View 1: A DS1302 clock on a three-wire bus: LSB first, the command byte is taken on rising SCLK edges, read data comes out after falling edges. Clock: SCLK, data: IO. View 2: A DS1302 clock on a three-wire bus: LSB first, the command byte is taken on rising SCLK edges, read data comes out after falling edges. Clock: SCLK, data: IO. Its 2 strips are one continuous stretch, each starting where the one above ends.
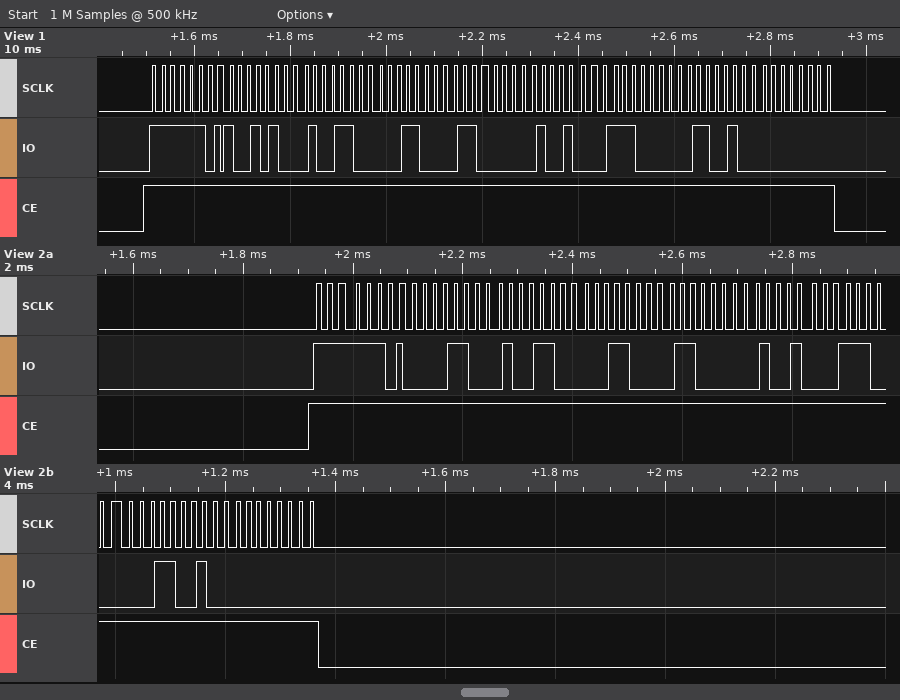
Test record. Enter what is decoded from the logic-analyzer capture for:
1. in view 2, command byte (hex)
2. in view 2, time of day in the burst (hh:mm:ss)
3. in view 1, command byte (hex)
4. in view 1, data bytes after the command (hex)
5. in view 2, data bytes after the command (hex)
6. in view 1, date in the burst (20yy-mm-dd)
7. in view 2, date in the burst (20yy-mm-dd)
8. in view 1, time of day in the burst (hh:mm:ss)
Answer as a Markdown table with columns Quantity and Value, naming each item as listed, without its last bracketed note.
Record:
| Quantity | Value |
|---|---|
| in view 2, command byte | 0xBF |
| in view 2, time of day in the burst | 18:32:30 |
| in view 1, command byte | 0xBF |
| in view 1, data bytes after the command | 29 32 18 06 12 07 26 00 |
| in view 2, data bytes after the command | 30 32 18 06 12 07 26 00 |
| in view 1, date in the burst | 2026-12-06 |
| in view 2, date in the burst | 2026-12-06 |
| in view 1, time of day in the burst | 18:32:29 |
